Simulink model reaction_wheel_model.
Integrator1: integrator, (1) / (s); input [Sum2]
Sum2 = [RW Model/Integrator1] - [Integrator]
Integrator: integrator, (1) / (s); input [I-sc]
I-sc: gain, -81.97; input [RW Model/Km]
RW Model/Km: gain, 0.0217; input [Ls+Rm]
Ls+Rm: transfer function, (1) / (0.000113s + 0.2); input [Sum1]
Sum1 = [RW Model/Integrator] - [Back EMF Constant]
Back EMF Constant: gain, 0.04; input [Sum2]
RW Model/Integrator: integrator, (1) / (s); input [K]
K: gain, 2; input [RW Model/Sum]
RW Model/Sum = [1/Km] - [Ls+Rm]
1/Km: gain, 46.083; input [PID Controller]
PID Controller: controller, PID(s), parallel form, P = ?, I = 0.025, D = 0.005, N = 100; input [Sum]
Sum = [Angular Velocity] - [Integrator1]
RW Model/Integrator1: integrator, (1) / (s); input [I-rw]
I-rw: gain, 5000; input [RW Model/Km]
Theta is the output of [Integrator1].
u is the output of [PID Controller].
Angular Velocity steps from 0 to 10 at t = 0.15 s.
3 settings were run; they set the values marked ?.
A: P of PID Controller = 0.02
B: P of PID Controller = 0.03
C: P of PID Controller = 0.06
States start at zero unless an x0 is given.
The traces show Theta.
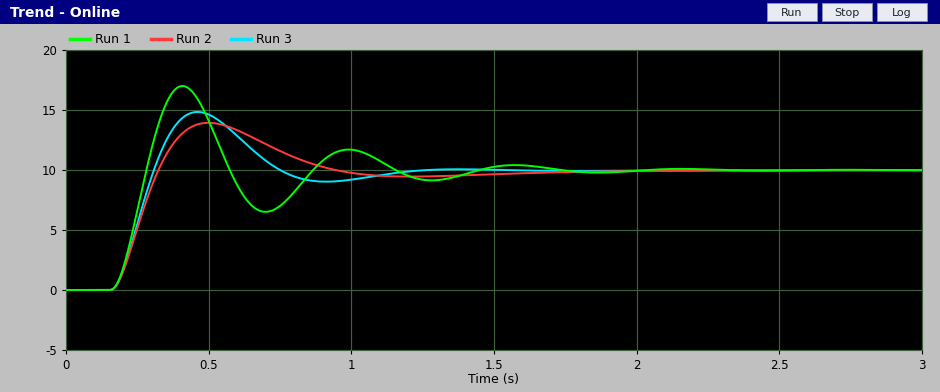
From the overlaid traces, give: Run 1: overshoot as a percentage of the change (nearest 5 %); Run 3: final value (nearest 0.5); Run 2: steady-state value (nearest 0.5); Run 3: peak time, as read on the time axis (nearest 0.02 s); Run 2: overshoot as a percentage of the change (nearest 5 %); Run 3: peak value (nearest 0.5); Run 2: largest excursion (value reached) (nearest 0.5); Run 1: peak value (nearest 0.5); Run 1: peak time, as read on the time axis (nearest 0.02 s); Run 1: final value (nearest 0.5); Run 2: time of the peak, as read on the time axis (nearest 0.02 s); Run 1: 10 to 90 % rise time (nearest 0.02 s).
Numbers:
70 %
10.0
10.0
0.46 s
40 %
15.0
14.0
17.0
0.40 s
10.0
0.50 s
0.08 s
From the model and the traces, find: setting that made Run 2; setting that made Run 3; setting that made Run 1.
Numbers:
A
B
C
